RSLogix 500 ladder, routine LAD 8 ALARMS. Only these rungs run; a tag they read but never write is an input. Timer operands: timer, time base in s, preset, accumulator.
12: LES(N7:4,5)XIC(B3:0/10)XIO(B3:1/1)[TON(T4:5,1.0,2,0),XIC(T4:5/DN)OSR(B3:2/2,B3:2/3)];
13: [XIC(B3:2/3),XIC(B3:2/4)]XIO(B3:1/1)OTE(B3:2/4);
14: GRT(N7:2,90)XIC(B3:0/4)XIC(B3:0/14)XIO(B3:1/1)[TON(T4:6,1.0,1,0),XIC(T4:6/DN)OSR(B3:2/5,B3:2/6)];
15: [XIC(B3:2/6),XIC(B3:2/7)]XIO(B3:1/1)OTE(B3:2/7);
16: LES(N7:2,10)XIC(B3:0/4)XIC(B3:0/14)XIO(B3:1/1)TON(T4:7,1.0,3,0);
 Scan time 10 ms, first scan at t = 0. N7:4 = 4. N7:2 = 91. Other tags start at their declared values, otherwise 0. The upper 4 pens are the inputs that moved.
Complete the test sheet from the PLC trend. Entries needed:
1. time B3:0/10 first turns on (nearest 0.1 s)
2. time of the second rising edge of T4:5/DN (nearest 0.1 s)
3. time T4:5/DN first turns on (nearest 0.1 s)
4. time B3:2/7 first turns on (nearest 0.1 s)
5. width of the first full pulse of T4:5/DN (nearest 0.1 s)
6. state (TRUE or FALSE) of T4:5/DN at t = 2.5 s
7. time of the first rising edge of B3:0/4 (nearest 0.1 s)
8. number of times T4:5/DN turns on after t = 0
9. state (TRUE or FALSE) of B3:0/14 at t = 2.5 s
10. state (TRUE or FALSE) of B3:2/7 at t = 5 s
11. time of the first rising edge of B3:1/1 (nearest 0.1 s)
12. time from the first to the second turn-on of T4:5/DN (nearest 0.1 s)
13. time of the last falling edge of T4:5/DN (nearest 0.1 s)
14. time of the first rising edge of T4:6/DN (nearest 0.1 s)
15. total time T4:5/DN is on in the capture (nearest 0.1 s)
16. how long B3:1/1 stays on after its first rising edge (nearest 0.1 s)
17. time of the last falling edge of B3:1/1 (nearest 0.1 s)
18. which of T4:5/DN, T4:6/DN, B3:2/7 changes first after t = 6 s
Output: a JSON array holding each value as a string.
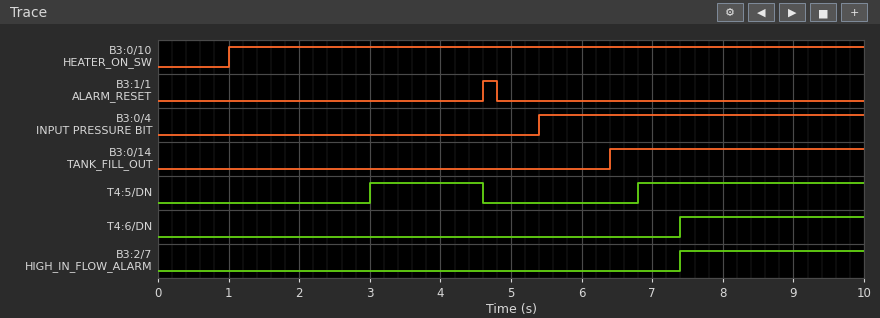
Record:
["1.0 s", "6.8 s", "3.0 s", "7.4 s", "1.6 s", "FALSE", "5.4 s", "2", "FALSE", "FALSE", "4.6 s", "3.8 s", "4.6 s", "7.4 s", "4.8 s", "0.2 s", "4.8 s", "T4:5/DN"]
